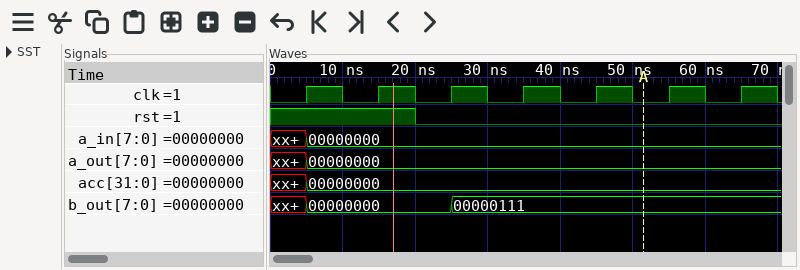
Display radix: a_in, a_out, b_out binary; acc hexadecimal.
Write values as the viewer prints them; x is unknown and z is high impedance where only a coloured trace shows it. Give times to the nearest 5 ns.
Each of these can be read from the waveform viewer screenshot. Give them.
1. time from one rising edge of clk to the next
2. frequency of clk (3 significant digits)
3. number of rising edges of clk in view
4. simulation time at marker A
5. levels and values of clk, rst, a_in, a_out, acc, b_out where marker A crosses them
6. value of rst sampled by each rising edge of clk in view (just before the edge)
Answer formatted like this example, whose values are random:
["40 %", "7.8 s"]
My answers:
["10 ns", "100 MHz", "7", "50 ns", "clk=0, rst=0, a_in=00000000, a_out=00000000, acc=00000000, b_out=00000111", "1 1 0 0 0 0 0"]
